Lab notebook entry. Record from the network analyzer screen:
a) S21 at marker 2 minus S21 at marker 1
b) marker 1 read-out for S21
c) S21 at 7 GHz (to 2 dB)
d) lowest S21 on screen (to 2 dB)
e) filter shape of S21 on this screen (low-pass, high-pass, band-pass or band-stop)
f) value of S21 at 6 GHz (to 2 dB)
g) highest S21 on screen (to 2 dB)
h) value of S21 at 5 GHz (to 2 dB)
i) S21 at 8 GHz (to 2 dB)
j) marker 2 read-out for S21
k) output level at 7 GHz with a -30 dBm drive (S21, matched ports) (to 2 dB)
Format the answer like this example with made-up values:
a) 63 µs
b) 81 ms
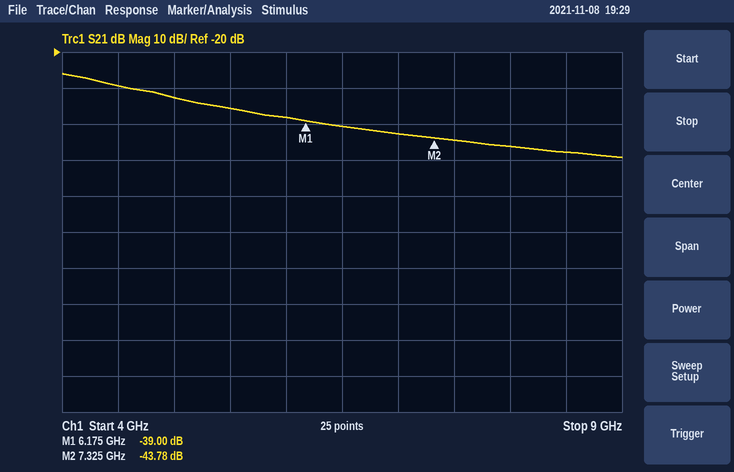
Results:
a) -4.78 dB
b) -39.00 dB
c) -42 dB
d) -50 dB
e) low-pass
f) -38 dB
g) -26 dB
h) -32 dB
i) -46 dB
j) -43.78 dB
k) -72 dBm
